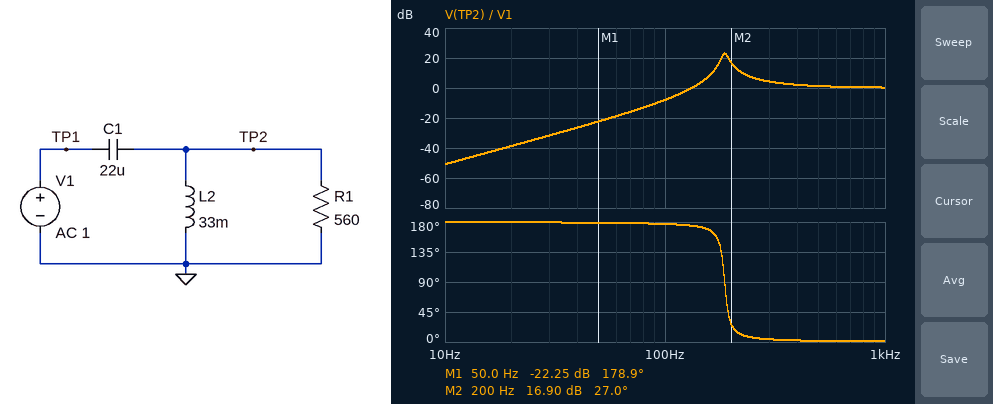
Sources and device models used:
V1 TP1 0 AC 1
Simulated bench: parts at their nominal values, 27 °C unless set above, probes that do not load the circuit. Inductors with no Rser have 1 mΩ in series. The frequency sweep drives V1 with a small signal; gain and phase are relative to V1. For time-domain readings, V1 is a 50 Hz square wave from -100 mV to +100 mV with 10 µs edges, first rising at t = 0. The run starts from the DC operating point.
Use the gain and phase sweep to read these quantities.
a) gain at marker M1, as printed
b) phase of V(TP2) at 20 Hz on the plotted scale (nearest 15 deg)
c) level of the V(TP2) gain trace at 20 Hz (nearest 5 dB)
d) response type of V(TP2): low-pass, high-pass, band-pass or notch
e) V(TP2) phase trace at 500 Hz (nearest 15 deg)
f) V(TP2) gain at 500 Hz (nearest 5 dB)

-22.25 dB
180 deg
-40 dB
high-pass
0 deg
0 dB
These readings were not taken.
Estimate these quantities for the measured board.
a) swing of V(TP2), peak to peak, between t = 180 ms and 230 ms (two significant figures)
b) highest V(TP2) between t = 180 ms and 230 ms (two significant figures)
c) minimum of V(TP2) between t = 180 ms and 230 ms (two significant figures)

240 mV
120 mV
-120 mV
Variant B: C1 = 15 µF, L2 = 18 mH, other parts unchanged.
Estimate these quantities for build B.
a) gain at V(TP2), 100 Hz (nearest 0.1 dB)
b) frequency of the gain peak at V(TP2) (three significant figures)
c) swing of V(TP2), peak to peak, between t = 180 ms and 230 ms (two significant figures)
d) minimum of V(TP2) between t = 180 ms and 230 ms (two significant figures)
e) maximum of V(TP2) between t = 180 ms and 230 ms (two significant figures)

-18.5 dB
307 Hz
260 mV
-130 mV
130 mV
